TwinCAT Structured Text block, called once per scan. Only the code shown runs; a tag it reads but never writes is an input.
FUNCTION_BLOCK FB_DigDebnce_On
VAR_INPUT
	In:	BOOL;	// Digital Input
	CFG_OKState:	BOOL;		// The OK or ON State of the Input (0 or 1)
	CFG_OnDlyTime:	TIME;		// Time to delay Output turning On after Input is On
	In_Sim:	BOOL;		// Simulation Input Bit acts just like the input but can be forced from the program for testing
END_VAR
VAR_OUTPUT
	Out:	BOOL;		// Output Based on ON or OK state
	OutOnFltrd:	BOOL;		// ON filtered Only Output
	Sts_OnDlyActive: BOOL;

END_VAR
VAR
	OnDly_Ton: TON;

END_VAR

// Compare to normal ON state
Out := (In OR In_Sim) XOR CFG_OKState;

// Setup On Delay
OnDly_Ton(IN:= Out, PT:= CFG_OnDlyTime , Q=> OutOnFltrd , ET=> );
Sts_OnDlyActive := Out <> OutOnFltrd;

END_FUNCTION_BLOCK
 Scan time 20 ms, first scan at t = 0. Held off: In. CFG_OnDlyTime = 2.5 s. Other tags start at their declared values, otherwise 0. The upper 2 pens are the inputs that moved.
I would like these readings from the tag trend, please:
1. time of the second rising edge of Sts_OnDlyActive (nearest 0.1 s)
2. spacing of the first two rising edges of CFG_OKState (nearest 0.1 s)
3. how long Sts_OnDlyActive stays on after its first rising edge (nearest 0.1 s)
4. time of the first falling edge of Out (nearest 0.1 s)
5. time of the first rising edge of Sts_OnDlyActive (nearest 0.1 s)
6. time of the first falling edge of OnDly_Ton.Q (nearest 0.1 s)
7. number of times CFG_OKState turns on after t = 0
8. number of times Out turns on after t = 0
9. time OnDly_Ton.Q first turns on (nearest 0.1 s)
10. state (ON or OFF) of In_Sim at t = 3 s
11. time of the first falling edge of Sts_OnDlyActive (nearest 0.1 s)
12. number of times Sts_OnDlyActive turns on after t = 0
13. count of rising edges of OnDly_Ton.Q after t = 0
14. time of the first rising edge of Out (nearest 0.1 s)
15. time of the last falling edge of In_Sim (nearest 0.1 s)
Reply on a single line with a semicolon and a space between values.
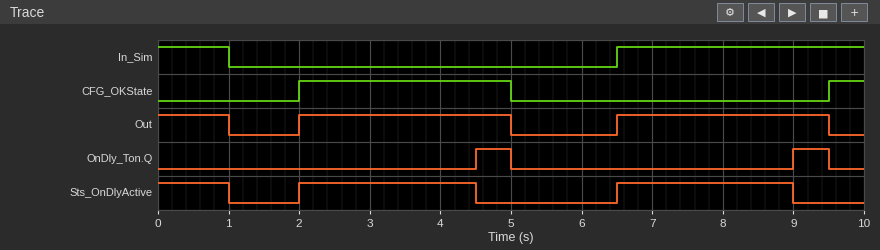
6.5 s; 7.5 s; 2.5 s; 1.0 s; 2.0 s; 5.0 s; 2; 2; 4.5 s; OFF; 1.0 s; 2; 2; 2.0 s; 1.0 s
